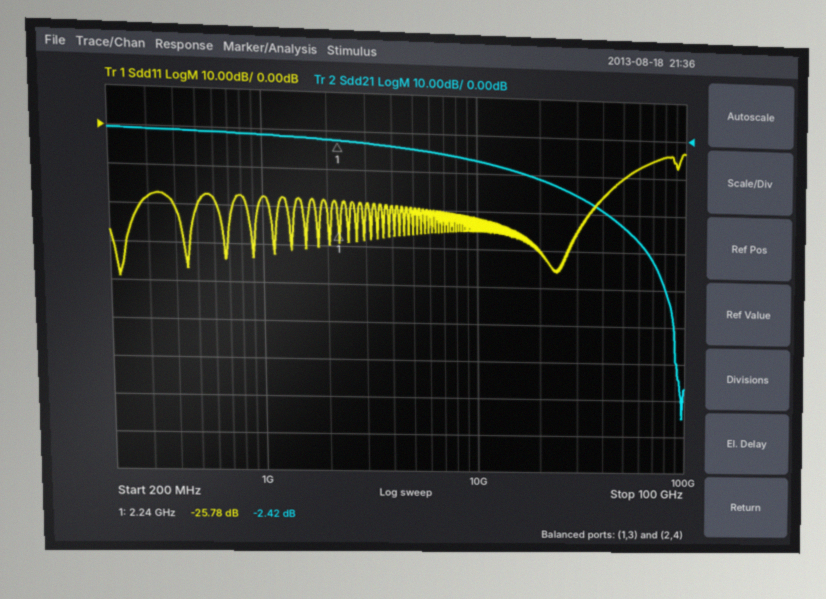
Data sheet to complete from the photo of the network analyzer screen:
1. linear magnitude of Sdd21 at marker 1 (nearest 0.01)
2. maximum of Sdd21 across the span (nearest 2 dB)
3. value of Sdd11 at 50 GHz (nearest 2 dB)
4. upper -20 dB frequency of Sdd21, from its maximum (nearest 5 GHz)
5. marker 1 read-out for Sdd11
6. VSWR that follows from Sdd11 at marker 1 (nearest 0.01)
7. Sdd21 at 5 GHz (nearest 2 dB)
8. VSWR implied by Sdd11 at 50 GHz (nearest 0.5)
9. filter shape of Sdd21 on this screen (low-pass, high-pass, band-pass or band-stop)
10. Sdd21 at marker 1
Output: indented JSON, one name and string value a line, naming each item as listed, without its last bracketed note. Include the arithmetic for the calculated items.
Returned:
{
  "linear magnitude of Sdd21 at marker 1": "10^(-2.42/20) ≈ 0.76",
  "maximum of Sdd21 across the span": "0 dB",
  "value of Sdd11 at 50 GHz": "-10 dB",
  "upper -20 dB frequency of Sdd21, from its maximum": "45 GHz",
  "marker 1 read-out for Sdd11": "-25.78 dB",
  "VSWR that follows from Sdd11 at marker 1": "(1 + 0.0514)/(1 − 0.0514) ≈ 1.11",
  "Sdd21 at 5 GHz": "-4 dB",
  "VSWR implied by Sdd11 at 50 GHz": "|Γ| = 10^(-10/20) = 0.3162; VSWR = (1 + 0.3162)/(1 − 0.3162) ≈ 1.92, so 2.0 to the nearest 0.5",
  "filter shape of Sdd21 on this screen": "low-pass",
  "Sdd21 at marker 1": "-2.42 dB"
}
